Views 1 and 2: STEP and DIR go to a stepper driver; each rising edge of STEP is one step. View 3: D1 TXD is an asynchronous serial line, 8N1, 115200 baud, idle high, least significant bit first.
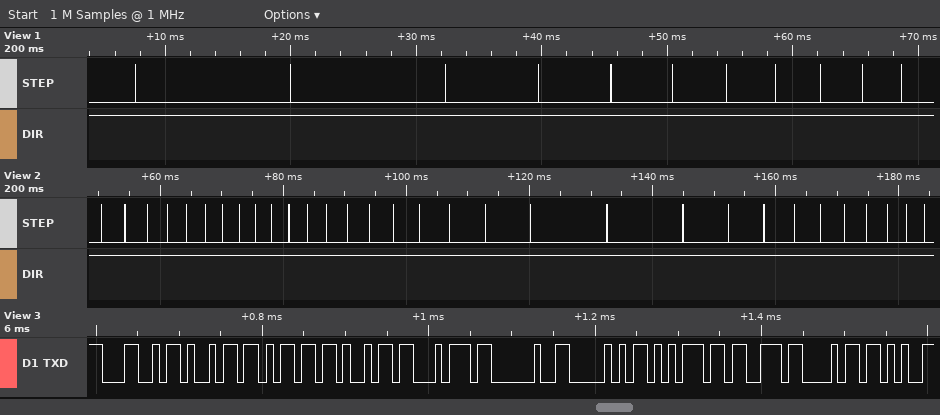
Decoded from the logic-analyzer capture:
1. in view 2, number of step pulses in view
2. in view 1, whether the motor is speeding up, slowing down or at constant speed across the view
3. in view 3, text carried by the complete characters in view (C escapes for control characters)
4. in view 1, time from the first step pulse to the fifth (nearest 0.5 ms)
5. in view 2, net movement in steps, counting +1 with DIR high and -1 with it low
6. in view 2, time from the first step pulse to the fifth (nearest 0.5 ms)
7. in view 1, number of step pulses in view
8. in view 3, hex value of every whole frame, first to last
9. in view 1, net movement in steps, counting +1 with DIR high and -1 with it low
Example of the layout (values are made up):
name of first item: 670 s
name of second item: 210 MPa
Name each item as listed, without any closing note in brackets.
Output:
in view 2, number of step pulses in view: 31
in view 1, whether the motor is speeding up, slowing down or at constant speed across the view: speeding up
in view 3, text carried by the complete characters in view: "Limit Push"
in view 1, time from the first step pulse to the fifth: 38.0 ms
in view 2, net movement in steps, counting +1 with DIR high and -1 with it low: +31
in view 2, time from the first step pulse to the fifth: 14.0 ms
in view 1, number of step pulses in view: 11
in view 3, hex value of every whole frame, first to last: 4C 69 6D 69 74 20 50 75 73 68
in view 1, net movement in steps, counting +1 with DIR high and -1 with it low: +11
